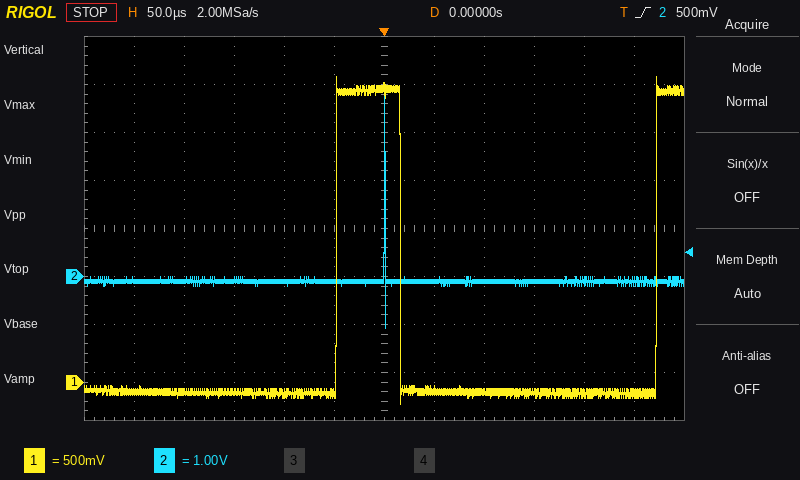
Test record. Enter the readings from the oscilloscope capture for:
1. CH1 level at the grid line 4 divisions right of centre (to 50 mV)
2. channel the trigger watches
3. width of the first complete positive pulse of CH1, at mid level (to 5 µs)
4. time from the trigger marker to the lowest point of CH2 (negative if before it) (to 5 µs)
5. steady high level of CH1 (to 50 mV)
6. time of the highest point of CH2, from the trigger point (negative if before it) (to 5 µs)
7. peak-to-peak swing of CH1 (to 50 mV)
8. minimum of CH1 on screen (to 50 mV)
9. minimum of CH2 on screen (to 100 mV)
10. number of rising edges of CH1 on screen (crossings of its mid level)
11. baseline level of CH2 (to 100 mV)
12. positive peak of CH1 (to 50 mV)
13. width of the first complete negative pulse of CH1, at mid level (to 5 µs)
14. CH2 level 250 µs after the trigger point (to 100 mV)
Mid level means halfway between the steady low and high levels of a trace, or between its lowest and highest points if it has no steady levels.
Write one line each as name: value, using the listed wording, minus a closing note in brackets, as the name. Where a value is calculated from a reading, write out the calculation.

CH1 level at the grid line 4 divisions right of centre: -100 mV
channel the trigger watches: CH2
width of the first complete positive pulse of CH1, at mid level: 65 µs
time from the trigger marker to the lowest point of CH2 (negative if before it): 0 µs
steady high level of CH1: 3.05 V
time of the highest point of CH2, from the trigger point (negative if before it): 0 µs
peak-to-peak swing of CH1: 3.20 V − (-200 mV) = 3.40 V
minimum of CH1 on screen: -200 mV
minimum of CH2 on screen: -1.1 V
number of rising edges of CH1 on screen: 2
baseline level of CH2: -100 mV
positive peak of CH1: 3.20 V
width of the first complete negative pulse of CH1, at mid level: 255 µs
CH2 level 250 µs after the trigger point: -100 mV
